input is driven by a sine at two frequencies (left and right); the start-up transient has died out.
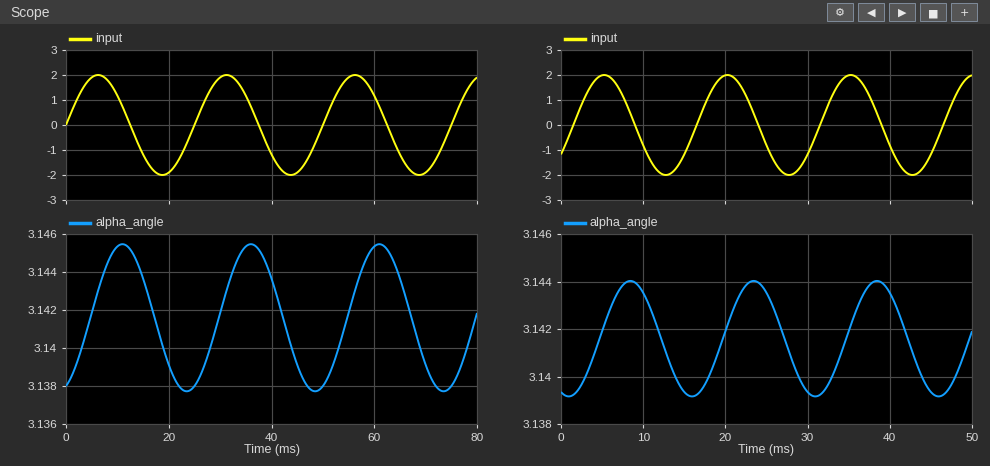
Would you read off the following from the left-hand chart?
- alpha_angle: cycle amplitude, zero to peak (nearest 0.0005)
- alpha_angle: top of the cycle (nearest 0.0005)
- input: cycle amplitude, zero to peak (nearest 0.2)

0.0040
3.1455
2.0
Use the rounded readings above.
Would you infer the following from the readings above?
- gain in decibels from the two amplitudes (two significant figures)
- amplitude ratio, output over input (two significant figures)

-54 dB
0.0020
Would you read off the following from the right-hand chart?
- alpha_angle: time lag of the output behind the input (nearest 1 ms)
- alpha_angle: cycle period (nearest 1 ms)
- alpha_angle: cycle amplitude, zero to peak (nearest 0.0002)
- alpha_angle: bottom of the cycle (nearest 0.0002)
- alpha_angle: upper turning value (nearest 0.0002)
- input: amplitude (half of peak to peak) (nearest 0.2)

3 ms
15 ms
0.0024
3.1392
3.1440
2.0
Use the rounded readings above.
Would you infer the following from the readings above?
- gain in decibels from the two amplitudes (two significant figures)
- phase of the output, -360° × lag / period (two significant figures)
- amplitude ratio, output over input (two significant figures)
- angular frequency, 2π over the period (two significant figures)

-58 dB
-72°
0.0012
0.42 rad/ms
